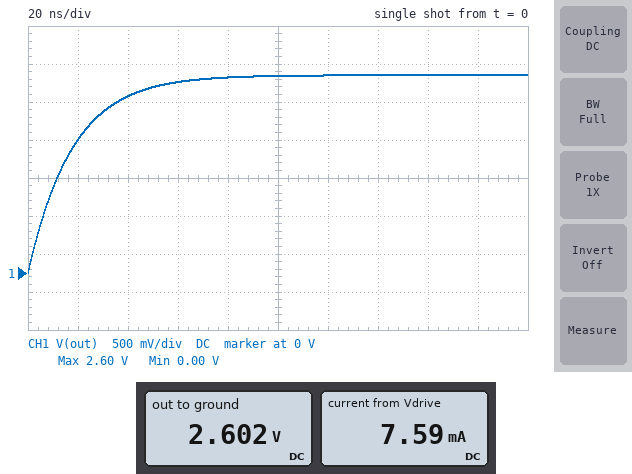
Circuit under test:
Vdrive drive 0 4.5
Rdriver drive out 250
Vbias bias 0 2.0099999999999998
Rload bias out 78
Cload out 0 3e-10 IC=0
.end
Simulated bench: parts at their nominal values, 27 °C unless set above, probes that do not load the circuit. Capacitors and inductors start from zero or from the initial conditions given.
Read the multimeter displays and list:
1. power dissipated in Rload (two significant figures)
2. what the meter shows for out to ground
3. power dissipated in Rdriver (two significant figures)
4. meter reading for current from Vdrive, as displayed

4.5 mW
2.602 V
14 mW
7.59 mA
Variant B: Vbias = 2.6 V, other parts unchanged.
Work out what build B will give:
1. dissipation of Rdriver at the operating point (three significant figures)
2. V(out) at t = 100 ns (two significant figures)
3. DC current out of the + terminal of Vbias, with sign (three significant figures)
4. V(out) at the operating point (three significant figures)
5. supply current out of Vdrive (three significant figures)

8.39 mW
3.0 V
-5.79 mA
3.05 V
5.79 mA
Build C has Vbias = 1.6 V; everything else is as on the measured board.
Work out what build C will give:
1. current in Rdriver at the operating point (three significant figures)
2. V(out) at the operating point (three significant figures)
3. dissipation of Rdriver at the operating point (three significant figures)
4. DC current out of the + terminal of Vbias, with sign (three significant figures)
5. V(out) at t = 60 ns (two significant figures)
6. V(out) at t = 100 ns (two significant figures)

8.84 mA
2.29 V
19.5 mW
-8.84 mA
2.2 V
2.3 V
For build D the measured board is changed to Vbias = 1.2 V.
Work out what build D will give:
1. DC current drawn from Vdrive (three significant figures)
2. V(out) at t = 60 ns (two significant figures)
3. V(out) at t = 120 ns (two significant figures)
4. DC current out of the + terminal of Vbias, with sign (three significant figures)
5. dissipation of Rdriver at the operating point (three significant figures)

10.1 mA
1.9 V
2.0 V
-10.1 mA
25.3 mW
